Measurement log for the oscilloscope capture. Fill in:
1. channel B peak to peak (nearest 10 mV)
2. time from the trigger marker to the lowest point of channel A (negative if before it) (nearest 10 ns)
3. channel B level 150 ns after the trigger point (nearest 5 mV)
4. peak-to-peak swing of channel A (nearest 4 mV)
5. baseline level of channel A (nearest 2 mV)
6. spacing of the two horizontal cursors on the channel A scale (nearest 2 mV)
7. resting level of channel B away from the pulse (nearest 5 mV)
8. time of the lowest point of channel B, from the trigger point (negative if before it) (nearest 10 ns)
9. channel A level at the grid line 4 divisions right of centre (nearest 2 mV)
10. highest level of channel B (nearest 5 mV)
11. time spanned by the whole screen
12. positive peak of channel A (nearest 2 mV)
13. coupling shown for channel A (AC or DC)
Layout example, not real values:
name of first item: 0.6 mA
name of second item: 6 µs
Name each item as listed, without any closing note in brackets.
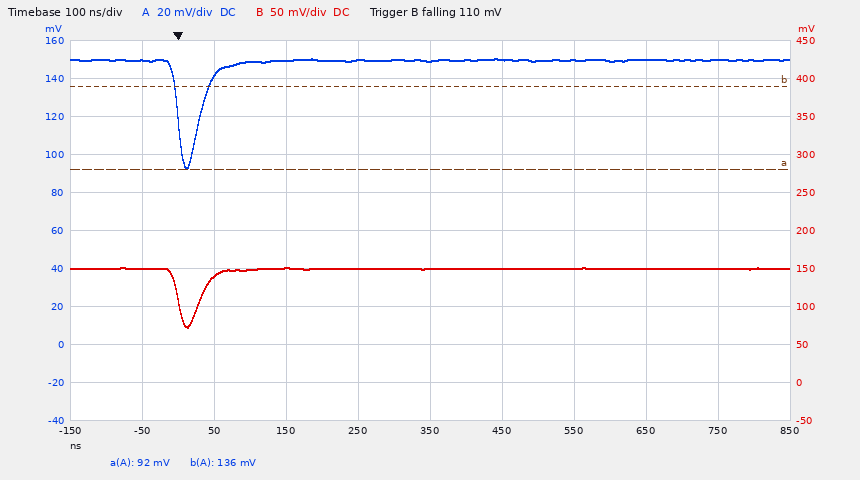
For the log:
channel B peak to peak: 80 mV
time from the trigger marker to the lowest point of channel A (negative if before it): +10 ns
channel B level 150 ns after the trigger point: 150 mV
peak-to-peak swing of channel A: 56 mV
baseline level of channel A: 150 mV
spacing of the two horizontal cursors on the channel A scale: 44 mV
resting level of channel B away from the pulse: 150 mV
time of the lowest point of channel B, from the trigger point (negative if before it): +10 ns
channel A level at the grid line 4 divisions right of centre: 150 mV
highest level of channel B: 150 mV
time spanned by the whole screen: 1 µs
positive peak of channel A: 150 mV
coupling shown for channel A: DC
